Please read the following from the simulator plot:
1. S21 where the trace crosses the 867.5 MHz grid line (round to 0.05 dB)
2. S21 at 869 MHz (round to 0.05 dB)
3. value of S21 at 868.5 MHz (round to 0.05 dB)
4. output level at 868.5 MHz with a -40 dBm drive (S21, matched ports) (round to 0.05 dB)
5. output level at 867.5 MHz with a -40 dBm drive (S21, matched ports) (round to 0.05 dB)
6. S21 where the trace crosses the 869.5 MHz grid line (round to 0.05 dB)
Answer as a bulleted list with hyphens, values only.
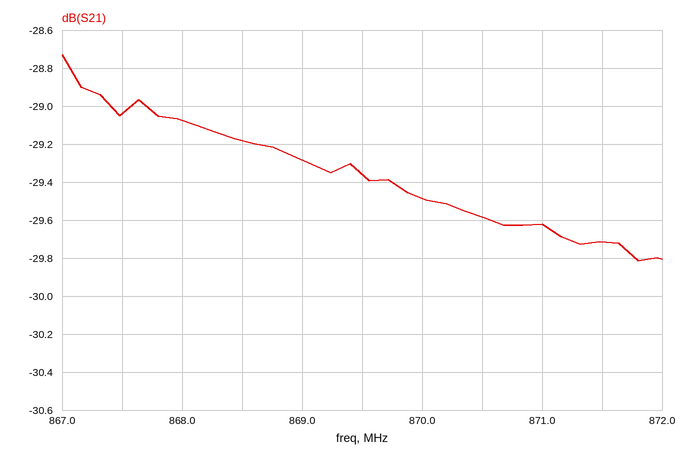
- -29.05 dB
- -29.30 dB
- -29.20 dB
- -69.20 dBm
- -69.05 dBm
- -29.35 dB
